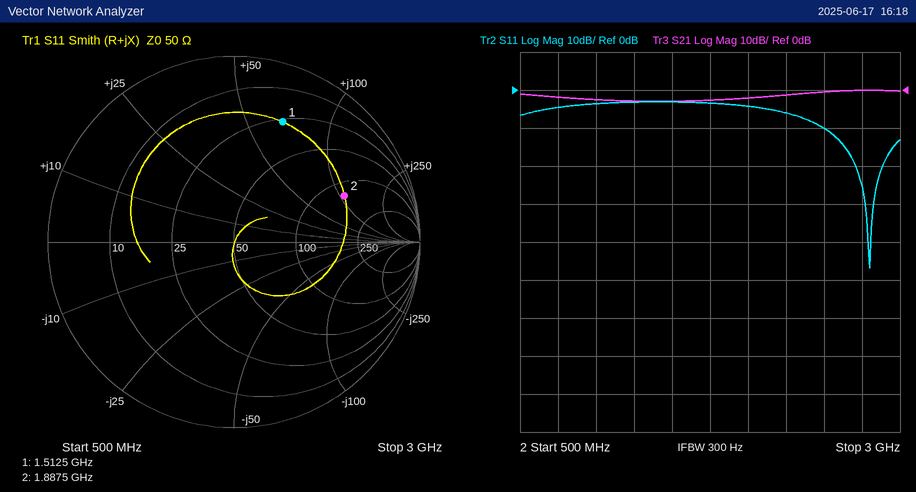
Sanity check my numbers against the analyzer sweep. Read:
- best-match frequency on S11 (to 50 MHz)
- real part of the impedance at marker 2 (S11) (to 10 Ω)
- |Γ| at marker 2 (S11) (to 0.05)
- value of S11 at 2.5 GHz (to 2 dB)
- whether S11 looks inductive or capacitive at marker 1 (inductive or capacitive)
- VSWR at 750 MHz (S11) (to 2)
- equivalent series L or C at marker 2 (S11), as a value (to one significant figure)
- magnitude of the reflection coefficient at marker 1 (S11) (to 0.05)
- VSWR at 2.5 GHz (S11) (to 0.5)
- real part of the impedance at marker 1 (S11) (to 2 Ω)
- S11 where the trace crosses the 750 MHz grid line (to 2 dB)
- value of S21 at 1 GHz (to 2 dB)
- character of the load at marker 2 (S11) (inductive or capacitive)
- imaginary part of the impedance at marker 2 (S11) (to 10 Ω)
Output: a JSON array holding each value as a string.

["2.80 GHz", "130 Ω", "0.65", "-10 dB", "inductive", "4", "9 nH", "0.70", "2.0", "26 Ω", "-4 dB", "-2 dB", "inductive", "+110 Ω"]
